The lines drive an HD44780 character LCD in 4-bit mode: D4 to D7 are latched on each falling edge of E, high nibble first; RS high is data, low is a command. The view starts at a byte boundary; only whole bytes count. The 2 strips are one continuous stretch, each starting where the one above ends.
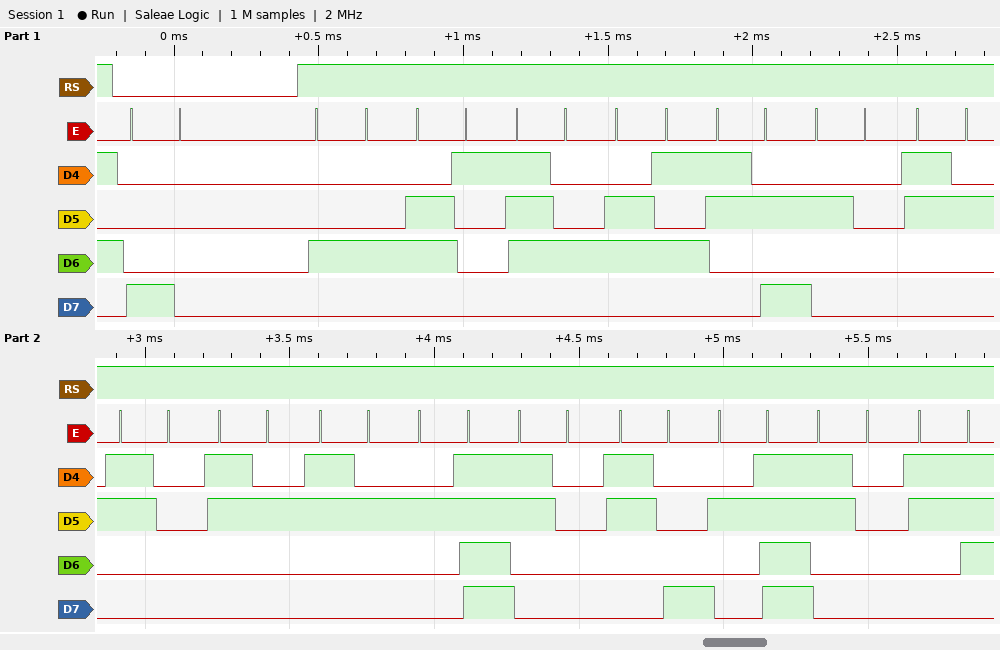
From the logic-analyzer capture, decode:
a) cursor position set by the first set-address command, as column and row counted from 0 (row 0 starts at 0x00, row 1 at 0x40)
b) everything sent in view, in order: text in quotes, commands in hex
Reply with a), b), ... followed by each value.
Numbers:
a) column 0, row 0
b) 0x80 "Date: 2022/08/07"
